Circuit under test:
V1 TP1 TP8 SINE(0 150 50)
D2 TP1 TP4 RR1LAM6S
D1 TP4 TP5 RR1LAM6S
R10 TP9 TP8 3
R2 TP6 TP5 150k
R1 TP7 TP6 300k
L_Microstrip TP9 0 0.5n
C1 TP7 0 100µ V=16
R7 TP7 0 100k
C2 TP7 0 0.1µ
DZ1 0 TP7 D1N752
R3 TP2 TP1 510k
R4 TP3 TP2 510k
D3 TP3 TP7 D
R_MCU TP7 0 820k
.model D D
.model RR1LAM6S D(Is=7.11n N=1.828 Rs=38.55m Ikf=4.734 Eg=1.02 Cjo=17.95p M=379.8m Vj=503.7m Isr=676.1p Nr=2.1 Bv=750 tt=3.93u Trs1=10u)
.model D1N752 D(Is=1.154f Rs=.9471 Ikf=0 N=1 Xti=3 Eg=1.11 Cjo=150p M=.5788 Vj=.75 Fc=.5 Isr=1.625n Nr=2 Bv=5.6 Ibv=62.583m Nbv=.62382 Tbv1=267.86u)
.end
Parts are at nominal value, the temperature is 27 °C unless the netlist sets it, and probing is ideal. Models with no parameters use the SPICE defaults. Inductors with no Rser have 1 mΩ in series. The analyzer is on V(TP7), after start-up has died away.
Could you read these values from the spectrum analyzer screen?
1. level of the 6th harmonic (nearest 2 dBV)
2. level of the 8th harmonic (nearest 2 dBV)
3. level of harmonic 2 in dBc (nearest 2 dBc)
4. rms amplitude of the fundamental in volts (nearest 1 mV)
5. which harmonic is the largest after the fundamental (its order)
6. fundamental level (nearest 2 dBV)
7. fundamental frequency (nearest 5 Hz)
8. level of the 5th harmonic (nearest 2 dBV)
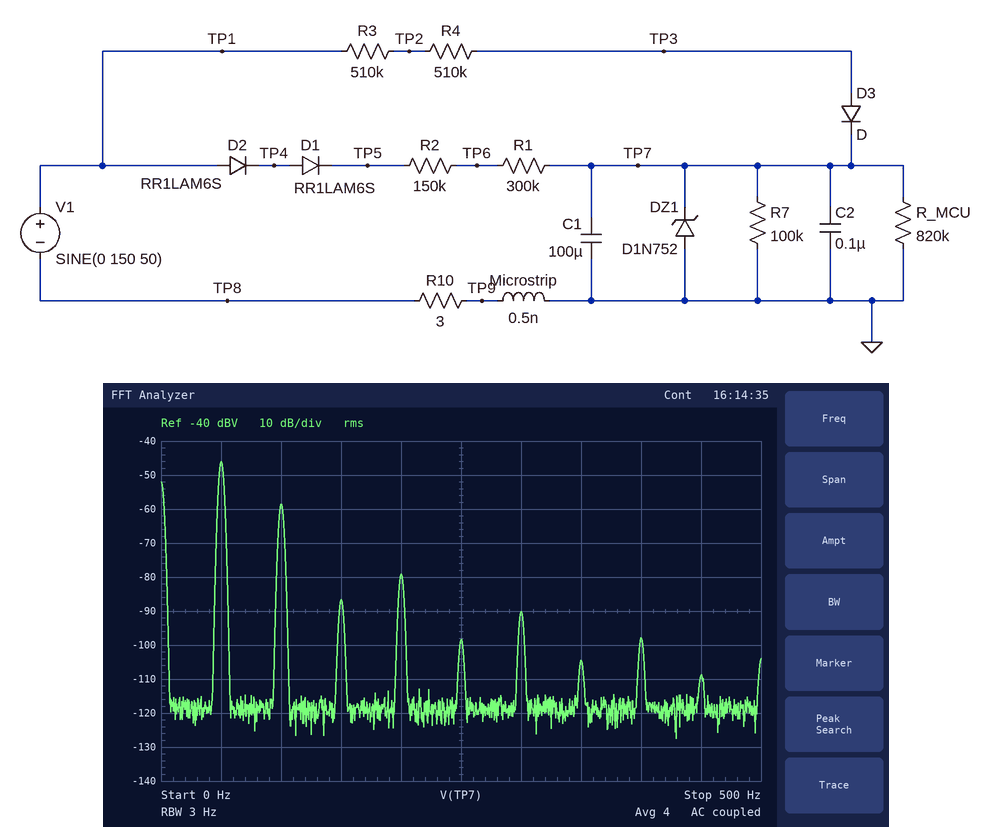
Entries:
-90 dBV
-98 dBV
-12 dBc
5 mV
2
-46 dBV
50 Hz
-98 dBV
